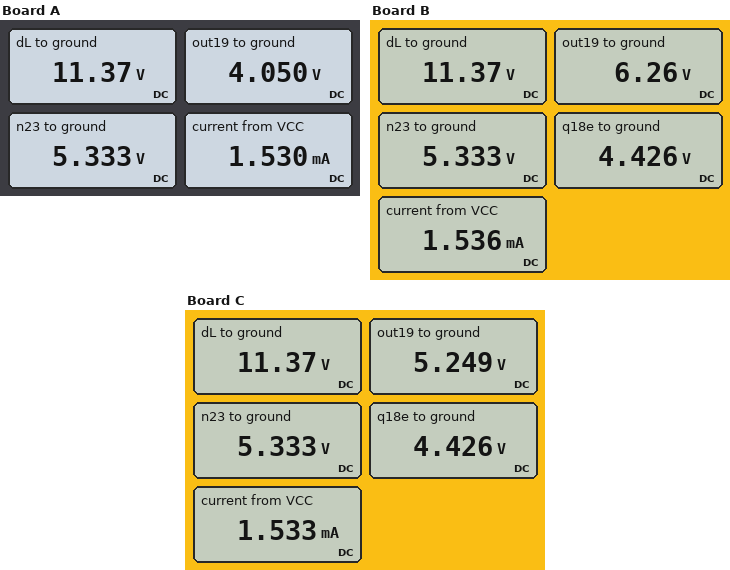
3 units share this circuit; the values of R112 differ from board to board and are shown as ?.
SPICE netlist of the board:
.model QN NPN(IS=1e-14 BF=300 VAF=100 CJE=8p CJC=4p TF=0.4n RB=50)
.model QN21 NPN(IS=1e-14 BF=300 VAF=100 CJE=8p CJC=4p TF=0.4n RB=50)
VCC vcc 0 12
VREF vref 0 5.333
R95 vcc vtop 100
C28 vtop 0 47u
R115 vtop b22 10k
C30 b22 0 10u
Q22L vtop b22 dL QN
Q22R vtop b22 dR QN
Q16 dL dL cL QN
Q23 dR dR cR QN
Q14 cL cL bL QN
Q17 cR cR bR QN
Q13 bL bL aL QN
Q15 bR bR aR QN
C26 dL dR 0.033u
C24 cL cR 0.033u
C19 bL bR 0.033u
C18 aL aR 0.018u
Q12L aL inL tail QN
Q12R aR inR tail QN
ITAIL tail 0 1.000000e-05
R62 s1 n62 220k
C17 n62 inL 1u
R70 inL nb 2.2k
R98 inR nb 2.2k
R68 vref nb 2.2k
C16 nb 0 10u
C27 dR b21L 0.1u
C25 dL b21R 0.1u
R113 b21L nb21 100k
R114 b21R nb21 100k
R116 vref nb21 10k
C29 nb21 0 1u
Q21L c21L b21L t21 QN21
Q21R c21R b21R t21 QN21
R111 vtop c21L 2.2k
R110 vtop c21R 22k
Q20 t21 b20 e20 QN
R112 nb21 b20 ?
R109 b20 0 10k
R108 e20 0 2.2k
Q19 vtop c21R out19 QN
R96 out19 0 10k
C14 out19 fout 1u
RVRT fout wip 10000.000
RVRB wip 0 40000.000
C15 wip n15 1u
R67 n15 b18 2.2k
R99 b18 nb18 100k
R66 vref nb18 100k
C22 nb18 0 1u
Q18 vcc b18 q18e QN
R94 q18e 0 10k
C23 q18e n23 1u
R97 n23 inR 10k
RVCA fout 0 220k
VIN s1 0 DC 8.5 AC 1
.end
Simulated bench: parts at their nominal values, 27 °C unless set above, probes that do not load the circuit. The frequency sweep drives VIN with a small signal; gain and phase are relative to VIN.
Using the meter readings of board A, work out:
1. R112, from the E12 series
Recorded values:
4.7 kΩ
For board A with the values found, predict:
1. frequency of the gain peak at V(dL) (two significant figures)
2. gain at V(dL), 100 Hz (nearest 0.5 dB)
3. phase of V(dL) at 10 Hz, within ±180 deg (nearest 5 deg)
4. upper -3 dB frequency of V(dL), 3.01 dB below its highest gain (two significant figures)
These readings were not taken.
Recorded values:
8.8 Hz
-70.0 dB
90 deg
10 Hz
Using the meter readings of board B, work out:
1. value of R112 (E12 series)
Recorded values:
12 kΩ
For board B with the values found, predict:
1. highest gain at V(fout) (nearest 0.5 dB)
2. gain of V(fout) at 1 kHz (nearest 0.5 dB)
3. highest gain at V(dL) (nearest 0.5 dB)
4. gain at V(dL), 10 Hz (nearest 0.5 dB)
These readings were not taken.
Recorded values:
-9.5 dB
-31.5 dB
-36.5 dB
-38.5 dB
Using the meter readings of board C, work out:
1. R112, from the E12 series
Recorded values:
8.2 kΩ
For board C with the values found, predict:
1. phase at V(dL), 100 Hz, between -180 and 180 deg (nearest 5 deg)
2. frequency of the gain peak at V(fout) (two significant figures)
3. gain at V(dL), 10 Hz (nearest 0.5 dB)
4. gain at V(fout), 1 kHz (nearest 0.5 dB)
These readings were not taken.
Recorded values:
130 deg
9.1 Hz
-38.0 dB
-29.5 dB
